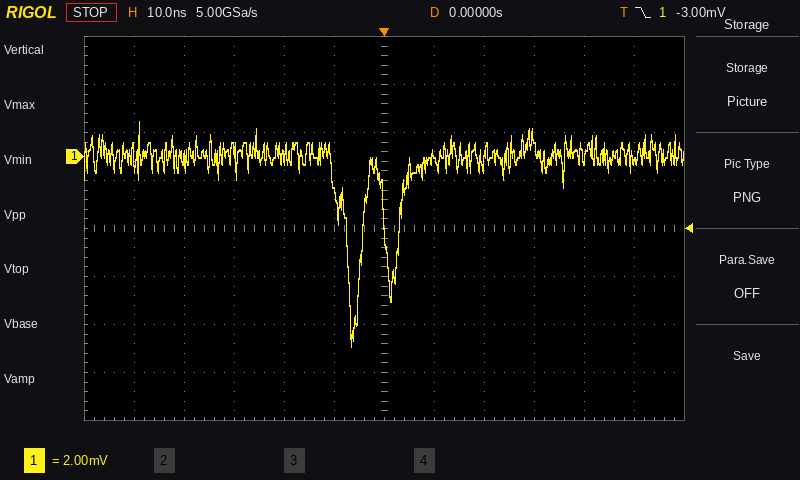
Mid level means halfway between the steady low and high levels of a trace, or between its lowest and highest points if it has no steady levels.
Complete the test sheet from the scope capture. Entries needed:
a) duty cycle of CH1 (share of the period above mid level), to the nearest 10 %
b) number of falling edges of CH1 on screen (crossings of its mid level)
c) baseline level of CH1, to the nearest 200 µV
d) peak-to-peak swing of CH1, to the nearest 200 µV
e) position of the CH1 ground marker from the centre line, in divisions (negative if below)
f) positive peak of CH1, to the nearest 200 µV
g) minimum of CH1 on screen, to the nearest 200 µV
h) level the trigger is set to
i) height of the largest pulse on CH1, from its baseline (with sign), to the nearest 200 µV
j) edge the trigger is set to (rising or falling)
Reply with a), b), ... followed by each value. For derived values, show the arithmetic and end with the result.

a) 60 %
b) 2
c) 0.0 mV
d) 1.4 mV − (-8.0 mV) = 9.4 mV
e) +1.5 div
f) 1.4 mV
g) -8.0 mV
h) -3.00 mV
i) -8.0 mV − (0.0 mV) = -8.0 mV
j) falling
